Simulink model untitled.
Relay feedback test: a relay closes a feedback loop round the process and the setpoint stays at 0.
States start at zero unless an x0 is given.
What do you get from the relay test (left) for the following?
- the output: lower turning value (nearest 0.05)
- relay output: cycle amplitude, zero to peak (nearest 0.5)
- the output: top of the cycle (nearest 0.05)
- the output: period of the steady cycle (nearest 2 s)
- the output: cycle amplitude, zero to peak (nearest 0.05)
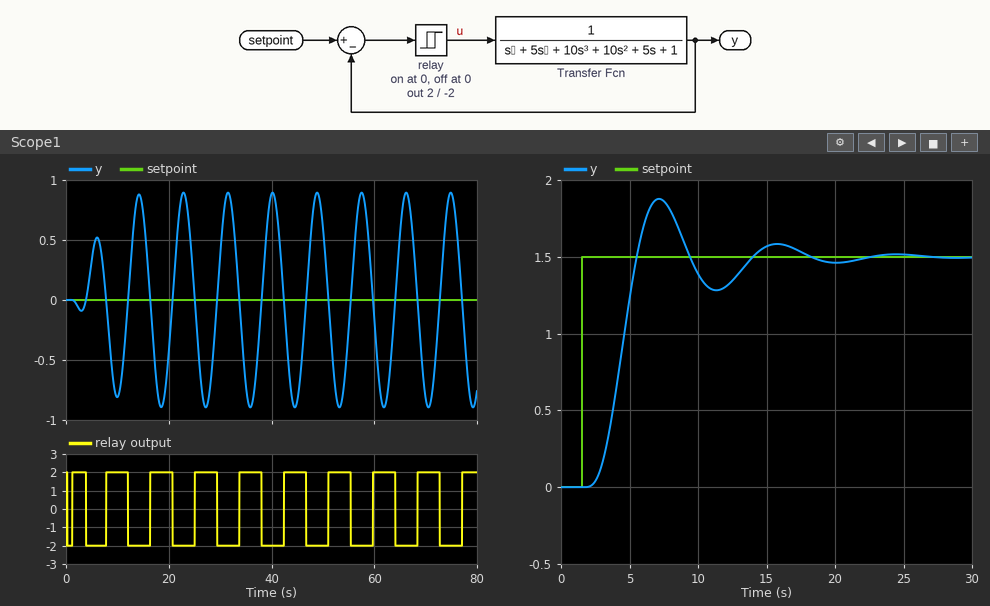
-0.90
2.0
0.90
8 s
0.90
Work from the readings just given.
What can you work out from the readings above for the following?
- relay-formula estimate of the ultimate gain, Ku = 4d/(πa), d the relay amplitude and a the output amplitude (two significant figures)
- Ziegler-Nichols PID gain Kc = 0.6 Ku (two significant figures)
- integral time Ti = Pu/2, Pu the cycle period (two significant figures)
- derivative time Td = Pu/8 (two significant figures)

2.8
1.7
4.0 s
1.0 s
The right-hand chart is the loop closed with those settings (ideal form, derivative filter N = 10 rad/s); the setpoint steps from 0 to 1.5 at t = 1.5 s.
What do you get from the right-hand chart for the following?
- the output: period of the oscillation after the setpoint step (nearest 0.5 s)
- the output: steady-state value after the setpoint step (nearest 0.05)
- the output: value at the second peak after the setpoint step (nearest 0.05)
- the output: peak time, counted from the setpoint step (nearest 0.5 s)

8.5 s
1.50
1.60
5.5 s
